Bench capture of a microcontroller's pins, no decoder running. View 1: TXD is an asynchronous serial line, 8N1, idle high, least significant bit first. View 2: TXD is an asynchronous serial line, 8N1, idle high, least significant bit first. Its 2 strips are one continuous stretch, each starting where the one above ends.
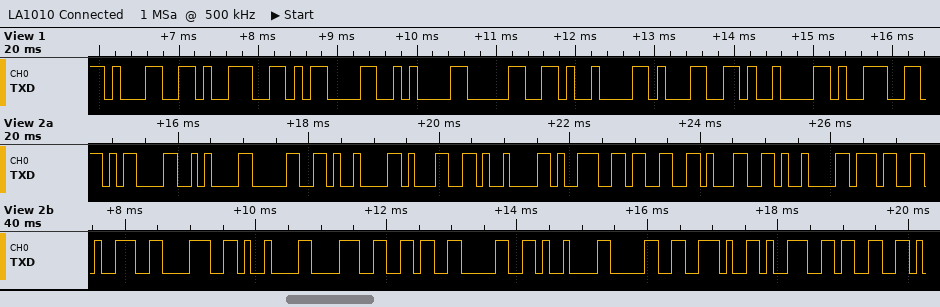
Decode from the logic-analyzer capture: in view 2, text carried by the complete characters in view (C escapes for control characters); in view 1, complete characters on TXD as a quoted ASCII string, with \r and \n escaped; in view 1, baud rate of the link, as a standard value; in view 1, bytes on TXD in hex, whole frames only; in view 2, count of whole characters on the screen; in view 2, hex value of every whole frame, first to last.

"\r\n0\t1\t931\t798\t860\t0.93"
"19\r\n0\t1\t9"
9600 baud
31 39 0D 0A 30 09 31 09 39
22
0D 0A 30 09 31 09 39 33 31 09 37 39 38 09 38 36 30 09 30 2E 39 33
